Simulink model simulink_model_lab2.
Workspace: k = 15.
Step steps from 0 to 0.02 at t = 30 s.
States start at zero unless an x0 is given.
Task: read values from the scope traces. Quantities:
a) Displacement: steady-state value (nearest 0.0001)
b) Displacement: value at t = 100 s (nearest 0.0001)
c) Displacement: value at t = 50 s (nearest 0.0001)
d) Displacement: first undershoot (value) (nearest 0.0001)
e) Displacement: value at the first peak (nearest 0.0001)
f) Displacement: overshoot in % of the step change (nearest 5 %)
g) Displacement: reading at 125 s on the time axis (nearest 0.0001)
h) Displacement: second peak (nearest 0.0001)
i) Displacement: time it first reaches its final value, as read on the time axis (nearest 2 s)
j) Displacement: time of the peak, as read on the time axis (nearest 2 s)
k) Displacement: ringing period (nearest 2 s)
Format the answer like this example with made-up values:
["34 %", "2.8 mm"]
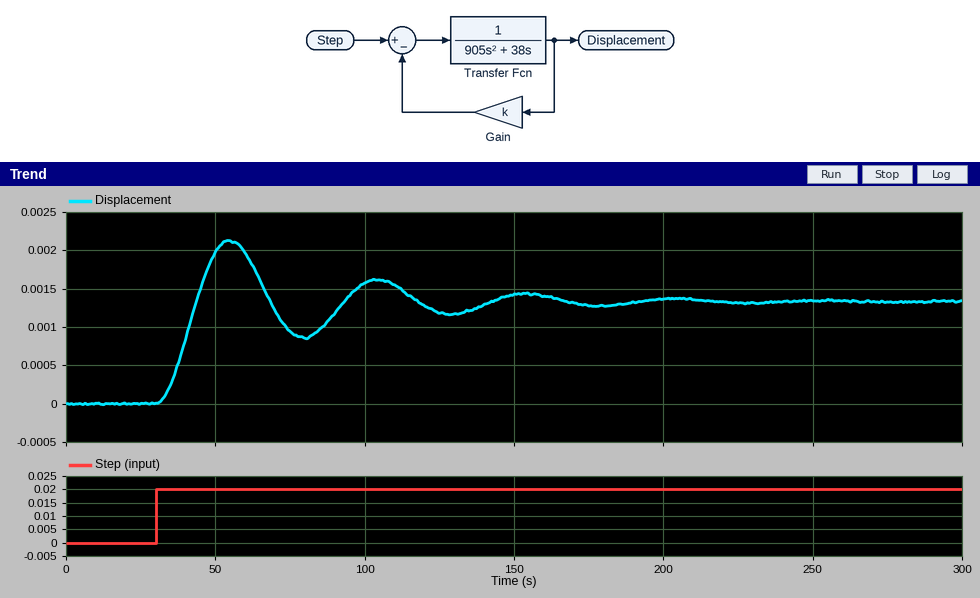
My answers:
["0.0013", "0.0016", "0.0020", "0.0009", "0.0021", "60 %", "0.0012", "0.0016", "44 s", "54 s", "50 s"]
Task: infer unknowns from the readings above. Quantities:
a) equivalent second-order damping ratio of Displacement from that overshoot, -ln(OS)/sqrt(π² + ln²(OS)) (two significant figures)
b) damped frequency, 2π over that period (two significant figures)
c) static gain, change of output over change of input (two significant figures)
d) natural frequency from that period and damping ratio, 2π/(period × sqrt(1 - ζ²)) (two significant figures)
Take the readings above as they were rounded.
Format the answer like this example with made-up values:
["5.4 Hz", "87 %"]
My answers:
["0.16", "0.13 rad/s", "0.065", "0.13 rad/s"]
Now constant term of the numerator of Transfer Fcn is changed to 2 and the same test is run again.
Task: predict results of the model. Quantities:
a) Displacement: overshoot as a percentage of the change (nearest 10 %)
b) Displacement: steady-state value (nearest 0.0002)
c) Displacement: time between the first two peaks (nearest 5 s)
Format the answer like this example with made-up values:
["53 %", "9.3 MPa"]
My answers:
["70 %", "0.0014", "35 s"]
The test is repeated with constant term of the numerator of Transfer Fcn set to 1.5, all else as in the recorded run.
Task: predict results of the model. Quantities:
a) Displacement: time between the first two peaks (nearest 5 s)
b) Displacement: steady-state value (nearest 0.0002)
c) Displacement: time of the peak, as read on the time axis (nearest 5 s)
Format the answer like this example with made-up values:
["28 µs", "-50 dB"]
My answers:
["40 s", "0.0014", "50 s"]
